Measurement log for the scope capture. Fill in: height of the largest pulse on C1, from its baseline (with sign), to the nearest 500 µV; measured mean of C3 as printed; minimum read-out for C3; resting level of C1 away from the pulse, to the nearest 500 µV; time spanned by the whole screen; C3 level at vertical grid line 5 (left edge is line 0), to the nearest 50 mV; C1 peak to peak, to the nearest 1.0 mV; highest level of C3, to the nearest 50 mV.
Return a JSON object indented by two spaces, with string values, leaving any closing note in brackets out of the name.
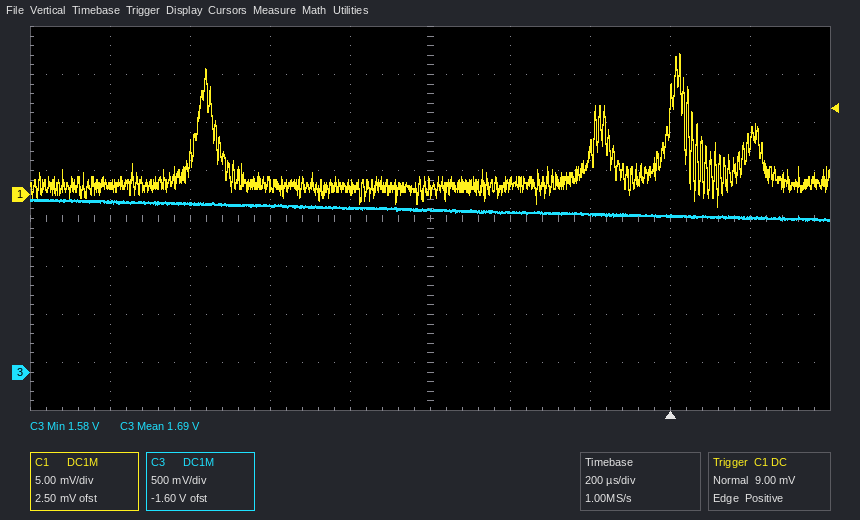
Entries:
{
  "height of the largest pulse on C1, from its baseline (with sign), to the nearest 500 µV": "+13.5 mV",
  "measured mean of C3 as printed": "1.69 V",
  "minimum read-out for C3": "1.58 V",
  "resting level of C1 away from the pulse, to the nearest 500 µV": "1.0 mV",
  "time spanned by the whole screen": "2 ms",
  "C3 level at vertical grid line 5 (left edge is line 0), to the nearest 50 mV": "1.70 V",
  "C1 peak to peak, to the nearest 1.0 mV": "16.0 mV",
  "highest level of C3, to the nearest 50 mV": "1.80 V"
}
